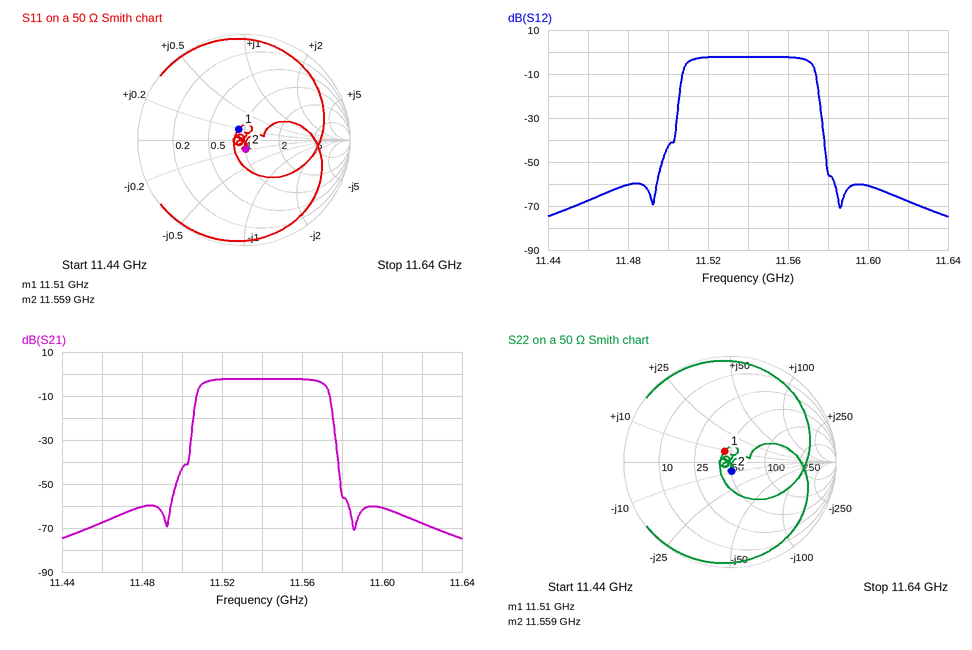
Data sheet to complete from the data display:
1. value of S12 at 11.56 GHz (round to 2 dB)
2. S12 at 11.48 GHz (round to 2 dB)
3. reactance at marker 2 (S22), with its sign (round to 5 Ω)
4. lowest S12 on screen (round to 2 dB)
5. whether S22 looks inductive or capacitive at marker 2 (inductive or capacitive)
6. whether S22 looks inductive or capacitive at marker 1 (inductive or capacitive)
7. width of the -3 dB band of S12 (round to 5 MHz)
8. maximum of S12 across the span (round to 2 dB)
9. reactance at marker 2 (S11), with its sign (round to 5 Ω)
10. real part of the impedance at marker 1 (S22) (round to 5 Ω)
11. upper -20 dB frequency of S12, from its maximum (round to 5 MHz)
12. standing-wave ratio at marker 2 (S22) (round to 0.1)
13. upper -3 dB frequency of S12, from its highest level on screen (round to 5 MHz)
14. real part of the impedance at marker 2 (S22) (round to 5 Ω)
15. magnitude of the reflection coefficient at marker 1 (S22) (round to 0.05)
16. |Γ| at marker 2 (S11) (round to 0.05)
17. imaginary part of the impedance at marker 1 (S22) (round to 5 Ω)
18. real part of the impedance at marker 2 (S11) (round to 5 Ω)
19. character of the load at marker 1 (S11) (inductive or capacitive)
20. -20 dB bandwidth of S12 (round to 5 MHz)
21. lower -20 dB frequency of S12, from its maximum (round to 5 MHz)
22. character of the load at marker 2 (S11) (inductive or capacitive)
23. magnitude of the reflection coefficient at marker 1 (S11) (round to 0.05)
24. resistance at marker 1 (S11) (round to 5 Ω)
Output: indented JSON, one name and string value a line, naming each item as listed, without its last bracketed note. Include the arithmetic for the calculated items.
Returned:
{
  "value of S12 at 11.56 GHz": "-2 dB",
  "S12 at 11.48 GHz": "-60 dB",
  "reactance at marker 2 (S22), with its sign": "-10 Ω",
  "lowest S12 on screen": "-74 dB",
  "whether S22 looks inductive or capacitive at marker 2": "capacitive",
  "whether S22 looks inductive or capacitive at marker 1": "inductive",
  "width of the -3 dB band of S12": "11.570 GHz − 11.510 GHz = 60 MHz",
  "maximum of S12 across the span": "-2 dB",
  "reactance at marker 2 (S11), with its sign": "-10 Ω",
  "real part of the impedance at marker 1 (S22)": "45 Ω",
  "upper -20 dB frequency of S12, from its maximum": "11.575 GHz",
  "standing-wave ratio at marker 2 (S22)": "1.2",
  "upper -3 dB frequency of S12, from its highest level on screen": "11.570 GHz",
  "real part of the impedance at marker 2 (S22)": "50 Ω",
  "magnitude of the reflection coefficient at marker 1 (S22)": "0.10",
  "|Γ| at marker 2 (S11)": "0.10",
  "imaginary part of the impedance at marker 1 (S22)": "+10 Ω",
  "real part of the impedance at marker 2 (S11)": "50 Ω",
  "character of the load at marker 1 (S11)": "inductive",
  "-20 dB bandwidth of S12": "11.575 GHz − 11.505 GHz = 70 MHz",
  "lower -20 dB frequency of S12, from its maximum": "11.505 GHz",
  "character of the load at marker 2 (S11)": "capacitive",
  "magnitude of the reflection coefficient at marker 1 (S11)": "0.10",
  "resistance at marker 1 (S11)": "45 Ω"
}
